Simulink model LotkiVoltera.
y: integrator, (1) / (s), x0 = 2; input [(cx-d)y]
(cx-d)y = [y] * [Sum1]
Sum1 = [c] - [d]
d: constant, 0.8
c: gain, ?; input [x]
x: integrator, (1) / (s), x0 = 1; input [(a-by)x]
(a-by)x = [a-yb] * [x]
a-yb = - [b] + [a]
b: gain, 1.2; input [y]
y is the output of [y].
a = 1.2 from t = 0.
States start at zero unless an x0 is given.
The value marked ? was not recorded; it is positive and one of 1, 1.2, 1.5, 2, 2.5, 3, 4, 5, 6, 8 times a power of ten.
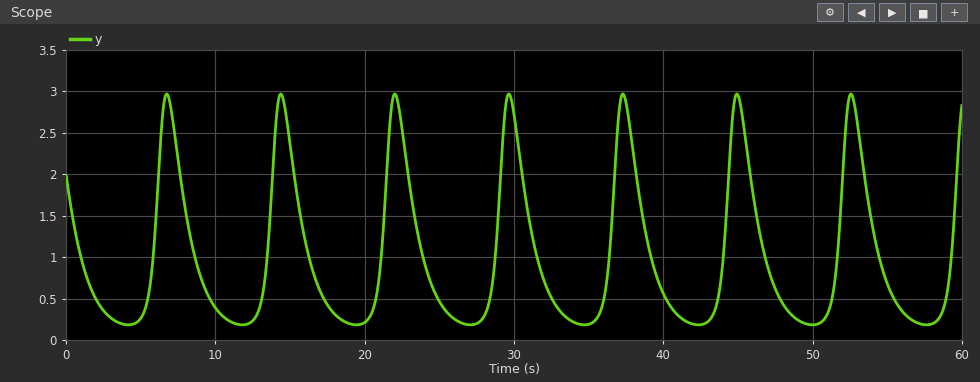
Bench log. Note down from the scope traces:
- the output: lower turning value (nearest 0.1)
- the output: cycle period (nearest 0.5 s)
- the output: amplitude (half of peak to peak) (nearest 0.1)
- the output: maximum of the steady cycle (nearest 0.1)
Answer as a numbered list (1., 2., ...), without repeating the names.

1. 0.2
2. 7.5 s
3. 1.4
4. 3.0
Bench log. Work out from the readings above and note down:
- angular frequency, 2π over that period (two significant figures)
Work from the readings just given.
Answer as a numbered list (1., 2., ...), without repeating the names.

1. 0.84 rad/s
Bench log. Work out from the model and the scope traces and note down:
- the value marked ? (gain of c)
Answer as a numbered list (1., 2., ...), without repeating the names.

1. 0.15
